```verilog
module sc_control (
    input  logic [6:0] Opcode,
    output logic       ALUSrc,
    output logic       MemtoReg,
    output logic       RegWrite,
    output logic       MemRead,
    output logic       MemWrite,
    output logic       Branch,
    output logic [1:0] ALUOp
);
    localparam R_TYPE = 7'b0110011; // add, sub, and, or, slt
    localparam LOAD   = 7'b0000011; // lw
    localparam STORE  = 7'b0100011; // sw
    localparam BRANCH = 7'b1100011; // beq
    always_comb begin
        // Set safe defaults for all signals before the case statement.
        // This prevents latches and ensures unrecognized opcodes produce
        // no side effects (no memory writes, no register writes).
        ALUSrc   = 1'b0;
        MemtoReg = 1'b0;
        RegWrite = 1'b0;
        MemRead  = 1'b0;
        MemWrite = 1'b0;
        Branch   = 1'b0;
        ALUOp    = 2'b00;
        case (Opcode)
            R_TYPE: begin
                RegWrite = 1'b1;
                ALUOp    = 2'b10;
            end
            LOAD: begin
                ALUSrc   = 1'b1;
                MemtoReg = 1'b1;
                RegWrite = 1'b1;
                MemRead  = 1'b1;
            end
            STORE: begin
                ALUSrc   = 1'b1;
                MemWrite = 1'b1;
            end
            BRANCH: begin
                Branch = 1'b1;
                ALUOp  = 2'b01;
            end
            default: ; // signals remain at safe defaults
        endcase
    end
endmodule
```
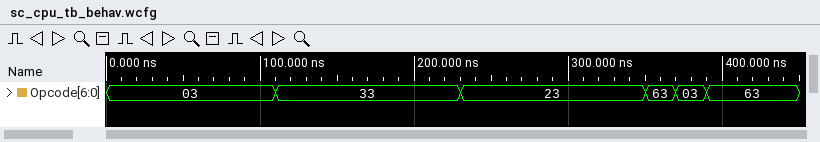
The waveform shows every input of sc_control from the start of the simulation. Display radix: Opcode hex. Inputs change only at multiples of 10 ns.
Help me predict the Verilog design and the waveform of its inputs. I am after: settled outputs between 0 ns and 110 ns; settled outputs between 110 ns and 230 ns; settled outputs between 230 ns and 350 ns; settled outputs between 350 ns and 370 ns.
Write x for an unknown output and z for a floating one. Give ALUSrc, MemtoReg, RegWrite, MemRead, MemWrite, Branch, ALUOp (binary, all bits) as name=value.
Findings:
ALUSrc=1, MemtoReg=1, RegWrite=1, MemRead=1, MemWrite=0, Branch=0, ALUOp=00
ALUSrc=0, MemtoReg=0, RegWrite=1, MemRead=0, MemWrite=0, Branch=0, ALUOp=10
ALUSrc=1, MemtoReg=0, RegWrite=0, MemRead=0, MemWrite=1, Branch=0, ALUOp=00
ALUSrc=0, MemtoReg=0, RegWrite=0, MemRead=0, MemWrite=0, Branch=1, ALUOp=01
